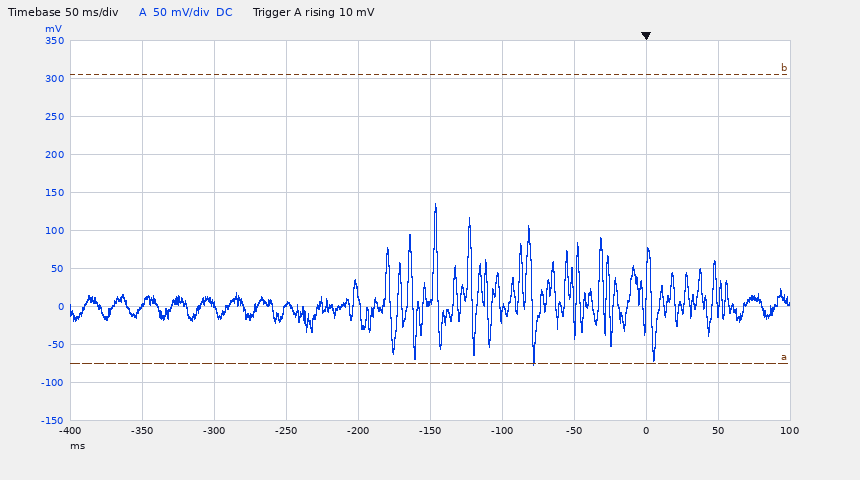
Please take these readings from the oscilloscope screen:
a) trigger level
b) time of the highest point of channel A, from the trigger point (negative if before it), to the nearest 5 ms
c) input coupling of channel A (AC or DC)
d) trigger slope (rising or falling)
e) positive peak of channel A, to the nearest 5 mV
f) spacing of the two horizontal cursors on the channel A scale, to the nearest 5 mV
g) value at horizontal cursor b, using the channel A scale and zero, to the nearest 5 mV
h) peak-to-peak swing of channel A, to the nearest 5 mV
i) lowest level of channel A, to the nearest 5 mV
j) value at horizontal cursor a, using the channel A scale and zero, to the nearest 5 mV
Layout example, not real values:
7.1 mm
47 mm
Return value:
10 mV
-145 ms
DC
rising
135 mV
380 mV
305 mV
210 mV
-75 mV
-75 mV
